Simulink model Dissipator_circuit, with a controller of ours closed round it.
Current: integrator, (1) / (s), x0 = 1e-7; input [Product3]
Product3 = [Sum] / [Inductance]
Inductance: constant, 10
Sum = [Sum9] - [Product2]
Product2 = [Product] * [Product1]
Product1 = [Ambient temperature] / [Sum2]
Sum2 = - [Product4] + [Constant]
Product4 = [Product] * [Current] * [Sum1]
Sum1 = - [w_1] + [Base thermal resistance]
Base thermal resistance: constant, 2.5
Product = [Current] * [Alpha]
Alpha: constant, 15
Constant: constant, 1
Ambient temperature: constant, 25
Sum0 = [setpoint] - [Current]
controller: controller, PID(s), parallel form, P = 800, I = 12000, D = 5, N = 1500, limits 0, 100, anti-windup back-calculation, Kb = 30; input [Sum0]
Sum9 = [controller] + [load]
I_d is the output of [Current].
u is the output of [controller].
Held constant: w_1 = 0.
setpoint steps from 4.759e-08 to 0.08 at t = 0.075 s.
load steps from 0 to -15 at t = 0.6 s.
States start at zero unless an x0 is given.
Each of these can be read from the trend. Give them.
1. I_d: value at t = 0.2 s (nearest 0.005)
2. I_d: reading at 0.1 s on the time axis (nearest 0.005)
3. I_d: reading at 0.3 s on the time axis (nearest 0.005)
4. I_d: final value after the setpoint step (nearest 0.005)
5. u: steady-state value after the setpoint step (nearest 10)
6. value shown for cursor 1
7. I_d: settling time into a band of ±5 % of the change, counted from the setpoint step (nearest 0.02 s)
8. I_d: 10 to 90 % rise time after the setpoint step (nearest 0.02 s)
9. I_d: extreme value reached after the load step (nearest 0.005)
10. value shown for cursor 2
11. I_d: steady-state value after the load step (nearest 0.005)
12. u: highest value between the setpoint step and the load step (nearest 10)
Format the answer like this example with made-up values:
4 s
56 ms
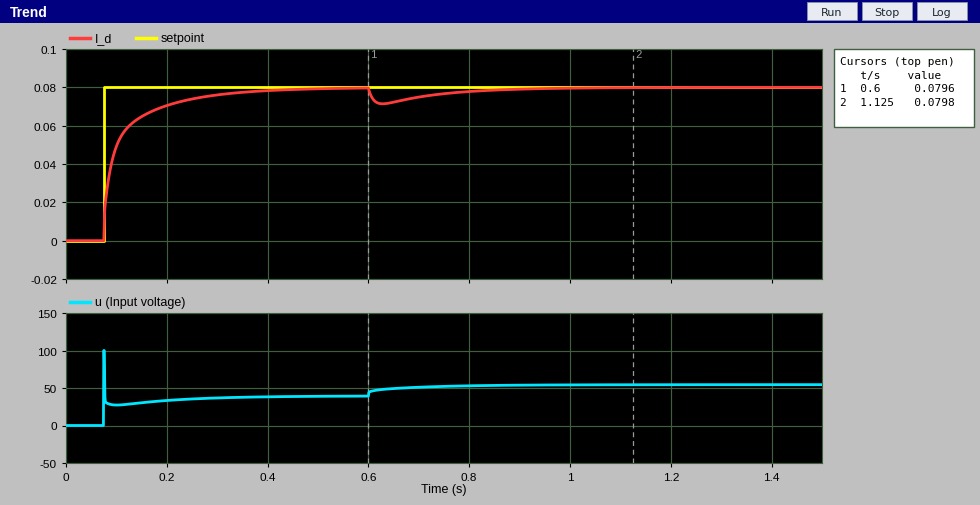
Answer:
0.070
0.050
0.075
0.080
40
0.0796
0.22 s
0.14 s
0.070
0.0798
0.080
100
